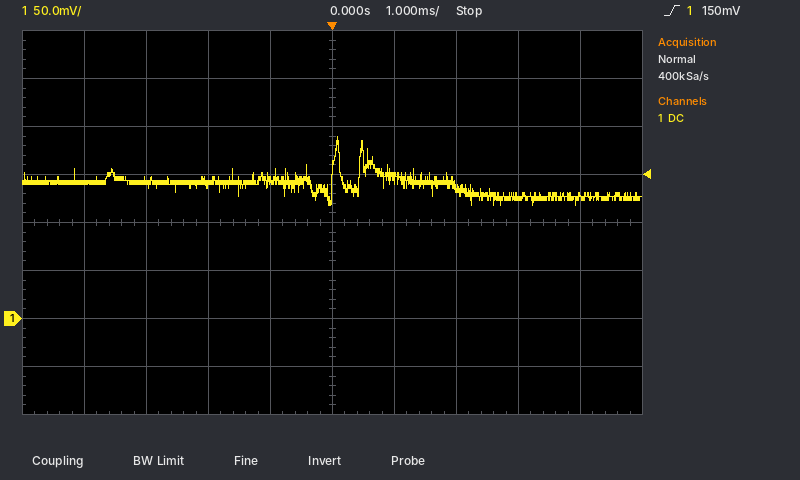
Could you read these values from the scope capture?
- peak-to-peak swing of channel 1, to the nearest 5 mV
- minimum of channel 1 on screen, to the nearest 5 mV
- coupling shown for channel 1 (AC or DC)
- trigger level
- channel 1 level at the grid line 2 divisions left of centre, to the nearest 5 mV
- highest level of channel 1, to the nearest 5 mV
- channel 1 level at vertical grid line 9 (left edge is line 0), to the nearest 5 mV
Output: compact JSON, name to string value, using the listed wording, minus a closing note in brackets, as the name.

{"peak-to-peak swing of channel 1, to the nearest 5 mV": "70 mV", "minimum of channel 1 on screen, to the nearest 5 mV": "120 mV", "coupling shown for channel 1": "DC", "trigger level": "150 mV", "channel 1 level at the grid line 2 divisions left of centre, to the nearest 5 mV": "140 mV", "highest level of channel 1, to the nearest 5 mV": "190 mV", "channel 1 level at vertical grid line 9 (left edge is line 0), to the nearest 5 mV": "125 mV"}
